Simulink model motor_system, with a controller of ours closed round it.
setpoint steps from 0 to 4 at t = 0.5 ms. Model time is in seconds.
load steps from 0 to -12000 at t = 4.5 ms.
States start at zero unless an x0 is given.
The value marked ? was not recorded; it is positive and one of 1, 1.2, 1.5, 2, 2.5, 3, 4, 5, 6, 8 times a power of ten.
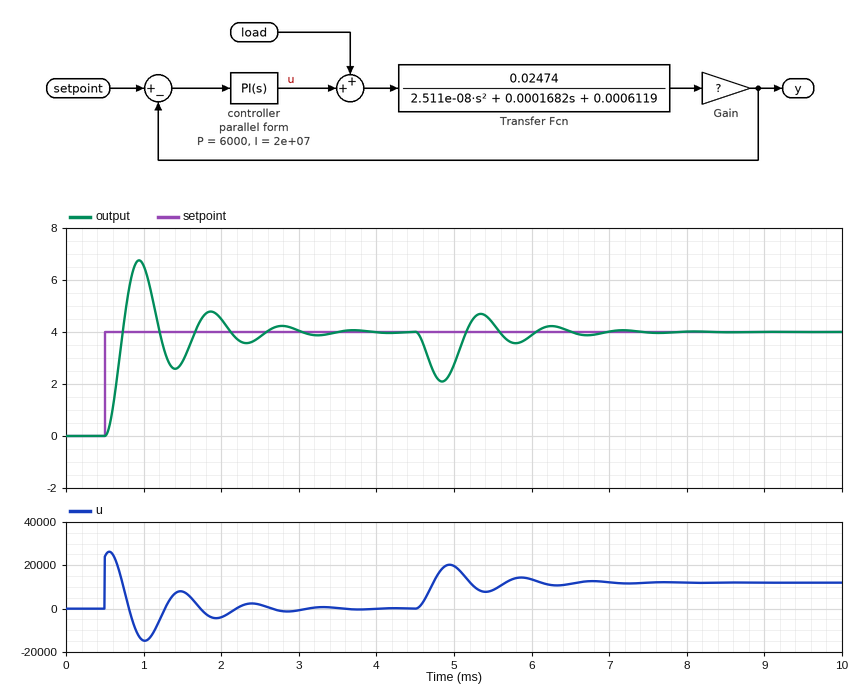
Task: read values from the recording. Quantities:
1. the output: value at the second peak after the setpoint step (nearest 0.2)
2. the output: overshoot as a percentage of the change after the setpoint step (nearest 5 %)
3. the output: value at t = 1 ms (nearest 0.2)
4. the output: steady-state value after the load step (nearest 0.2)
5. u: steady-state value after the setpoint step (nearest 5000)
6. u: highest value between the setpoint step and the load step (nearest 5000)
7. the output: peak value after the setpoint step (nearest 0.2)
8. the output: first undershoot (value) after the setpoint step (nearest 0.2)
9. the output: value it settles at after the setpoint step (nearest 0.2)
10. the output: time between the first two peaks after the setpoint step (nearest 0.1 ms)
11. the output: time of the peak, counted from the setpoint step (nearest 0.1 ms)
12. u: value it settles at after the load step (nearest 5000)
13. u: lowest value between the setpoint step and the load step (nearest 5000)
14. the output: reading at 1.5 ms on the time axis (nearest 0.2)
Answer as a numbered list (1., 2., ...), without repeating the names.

1. 4.8
2. 70 %
3. 6.6
4. 4.0
5. 0
6. 25000
7. 6.8
8. 2.6
9. 4.0
10. 0.9 ms
11. 0.4 ms
12. 10000
13. -15000
14. 2.8
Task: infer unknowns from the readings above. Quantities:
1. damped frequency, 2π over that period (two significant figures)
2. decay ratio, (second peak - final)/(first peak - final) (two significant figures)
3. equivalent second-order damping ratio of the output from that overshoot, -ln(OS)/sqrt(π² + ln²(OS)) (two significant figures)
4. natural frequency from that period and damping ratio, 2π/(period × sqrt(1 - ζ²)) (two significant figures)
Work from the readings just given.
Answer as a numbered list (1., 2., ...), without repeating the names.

1. 7.0 rad/ms
2. 0.29
3. 0.11
4. 7.0 rad/ms
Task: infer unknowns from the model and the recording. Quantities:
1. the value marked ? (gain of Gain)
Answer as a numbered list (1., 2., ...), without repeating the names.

1. 0.01
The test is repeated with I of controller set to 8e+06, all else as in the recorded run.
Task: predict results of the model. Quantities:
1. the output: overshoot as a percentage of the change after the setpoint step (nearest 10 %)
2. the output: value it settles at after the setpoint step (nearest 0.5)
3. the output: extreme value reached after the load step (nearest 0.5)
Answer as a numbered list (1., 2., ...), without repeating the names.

1. 40 %
2. 4.0
3. 2.0
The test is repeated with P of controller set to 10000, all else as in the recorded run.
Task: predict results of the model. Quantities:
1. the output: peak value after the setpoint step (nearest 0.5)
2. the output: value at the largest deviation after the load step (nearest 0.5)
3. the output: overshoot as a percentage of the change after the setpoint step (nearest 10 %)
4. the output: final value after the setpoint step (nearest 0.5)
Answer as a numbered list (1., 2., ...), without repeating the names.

1. 6.5
2. 2.5
3. 60 %
4. 4.0
